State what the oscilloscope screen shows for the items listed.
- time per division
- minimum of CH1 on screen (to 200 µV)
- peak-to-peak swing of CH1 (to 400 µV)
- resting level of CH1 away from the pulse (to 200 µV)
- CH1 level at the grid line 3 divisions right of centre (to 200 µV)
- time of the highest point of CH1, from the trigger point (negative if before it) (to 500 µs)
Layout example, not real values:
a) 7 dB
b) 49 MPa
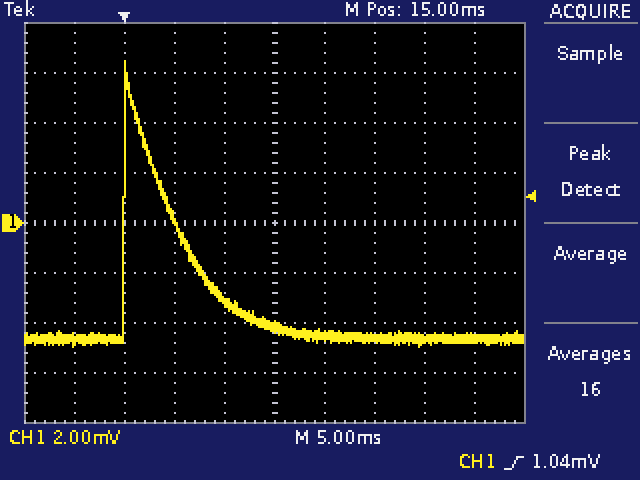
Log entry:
a) 5 ms
b) -5.0 mV
c) 11.6 mV
d) -4.6 mV
e) -4.6 mV
f) 0.0 ms
